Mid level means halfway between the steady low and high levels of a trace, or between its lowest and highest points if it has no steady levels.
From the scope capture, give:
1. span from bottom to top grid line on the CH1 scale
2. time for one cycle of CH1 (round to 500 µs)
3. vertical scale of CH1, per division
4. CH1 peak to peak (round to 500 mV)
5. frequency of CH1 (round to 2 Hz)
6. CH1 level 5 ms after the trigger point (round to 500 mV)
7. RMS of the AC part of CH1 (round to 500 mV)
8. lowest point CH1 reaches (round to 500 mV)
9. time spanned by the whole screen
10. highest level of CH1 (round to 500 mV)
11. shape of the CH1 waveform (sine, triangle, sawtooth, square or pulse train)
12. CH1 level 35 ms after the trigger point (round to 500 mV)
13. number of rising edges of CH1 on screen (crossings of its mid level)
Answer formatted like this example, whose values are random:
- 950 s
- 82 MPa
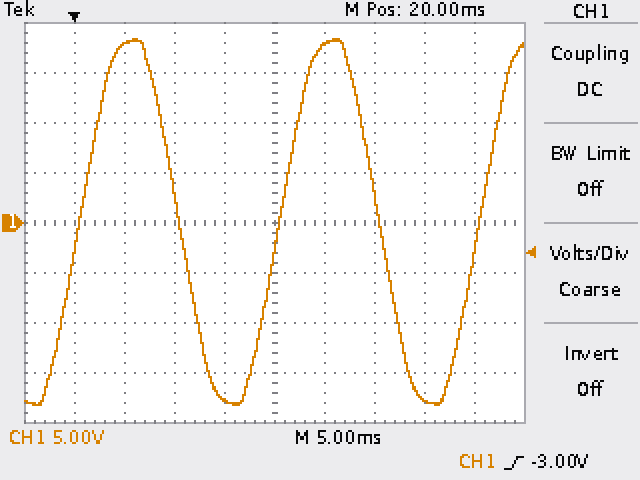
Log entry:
- 40 V
- 20.0 ms
- 5 V
- 36.5 V
- 50 Hz
- 18.0 V
- 13.0 V
- -18.0 V
- 50 ms
- 18.5 V
- sine
- -17.5 V
- 3
